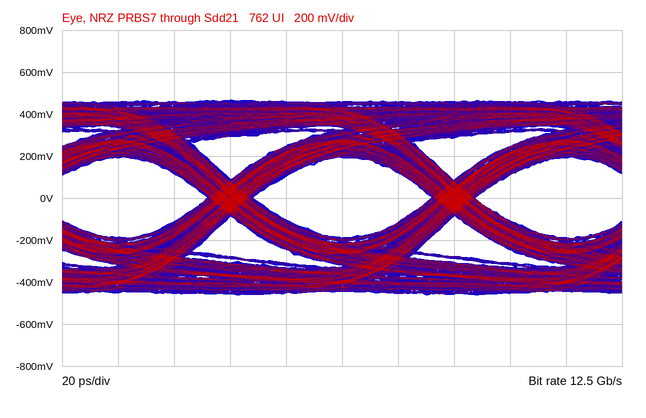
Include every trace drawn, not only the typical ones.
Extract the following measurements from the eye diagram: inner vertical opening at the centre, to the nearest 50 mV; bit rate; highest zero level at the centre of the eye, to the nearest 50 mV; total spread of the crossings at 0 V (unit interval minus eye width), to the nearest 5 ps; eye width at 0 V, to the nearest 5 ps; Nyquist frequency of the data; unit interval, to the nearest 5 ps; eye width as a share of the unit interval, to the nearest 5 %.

400 mV
12.5 Gb/s
-200 mV
15 ps
65 ps
6.25 GHz
80 ps
80 %
